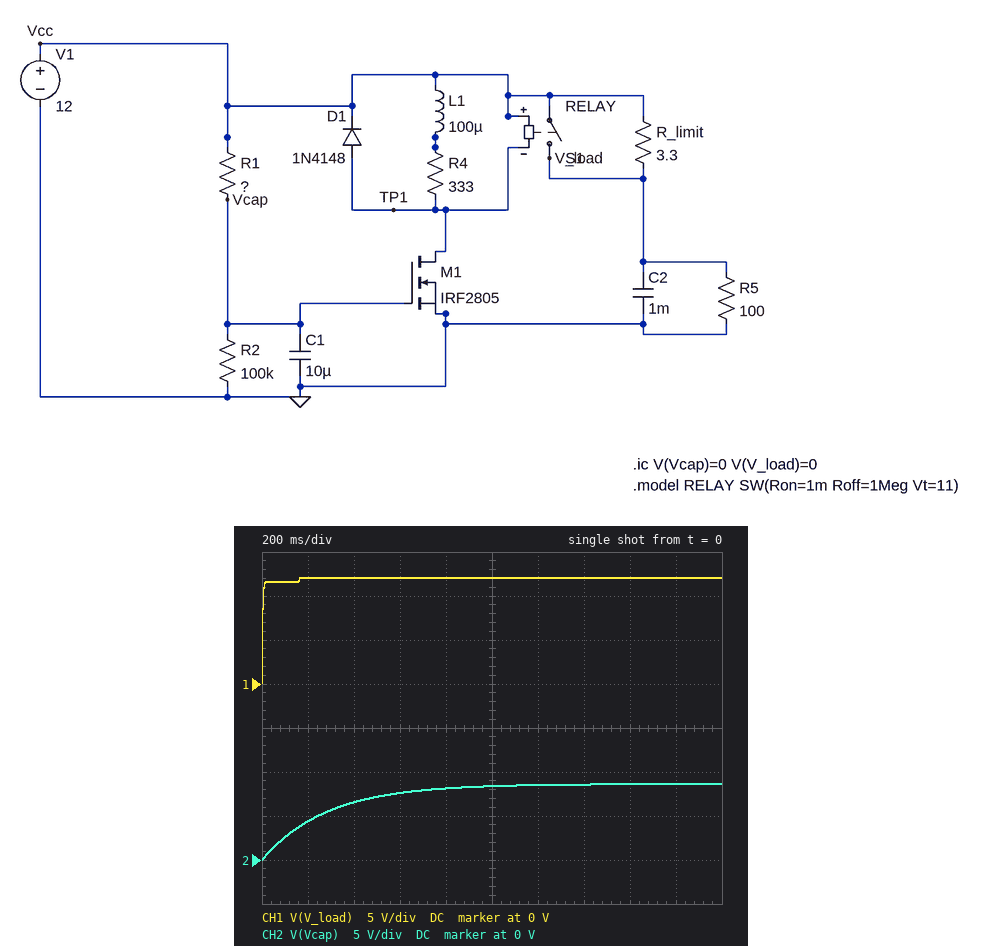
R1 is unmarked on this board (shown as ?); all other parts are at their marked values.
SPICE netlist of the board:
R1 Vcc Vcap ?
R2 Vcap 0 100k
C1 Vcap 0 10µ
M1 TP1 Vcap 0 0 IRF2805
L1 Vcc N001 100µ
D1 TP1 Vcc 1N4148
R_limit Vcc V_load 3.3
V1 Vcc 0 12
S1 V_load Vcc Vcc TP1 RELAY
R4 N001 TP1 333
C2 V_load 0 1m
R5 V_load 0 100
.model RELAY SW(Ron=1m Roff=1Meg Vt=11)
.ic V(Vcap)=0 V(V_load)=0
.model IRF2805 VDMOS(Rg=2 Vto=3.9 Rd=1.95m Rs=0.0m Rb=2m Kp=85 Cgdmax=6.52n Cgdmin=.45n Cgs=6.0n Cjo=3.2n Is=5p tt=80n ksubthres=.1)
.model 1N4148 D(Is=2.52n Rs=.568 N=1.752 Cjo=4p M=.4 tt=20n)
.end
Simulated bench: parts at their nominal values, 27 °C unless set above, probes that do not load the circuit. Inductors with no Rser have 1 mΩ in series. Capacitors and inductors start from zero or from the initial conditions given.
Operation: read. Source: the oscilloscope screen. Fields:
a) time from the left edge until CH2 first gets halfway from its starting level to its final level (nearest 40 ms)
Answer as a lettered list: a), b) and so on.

a) 200 ms
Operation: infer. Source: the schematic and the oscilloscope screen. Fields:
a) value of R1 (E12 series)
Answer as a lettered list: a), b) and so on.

a) 39 kΩ
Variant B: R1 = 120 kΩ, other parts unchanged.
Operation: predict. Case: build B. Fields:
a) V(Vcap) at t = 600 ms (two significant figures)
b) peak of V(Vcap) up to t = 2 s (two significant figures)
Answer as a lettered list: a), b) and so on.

a) 3.6 V
b) 5.3 V
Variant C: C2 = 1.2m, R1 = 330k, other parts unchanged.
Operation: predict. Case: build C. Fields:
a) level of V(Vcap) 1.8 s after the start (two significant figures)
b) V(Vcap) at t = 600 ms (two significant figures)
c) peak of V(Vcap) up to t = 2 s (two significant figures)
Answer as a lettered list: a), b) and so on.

a) 2.5 V
b) 1.5 V
c) 2.6 V
